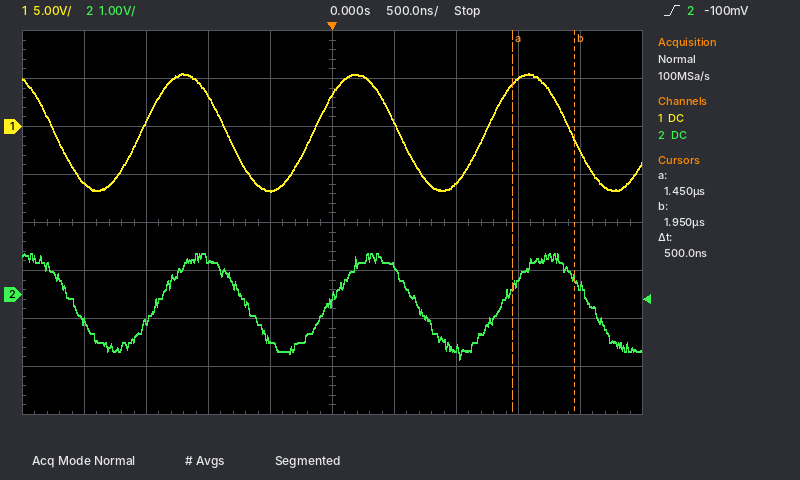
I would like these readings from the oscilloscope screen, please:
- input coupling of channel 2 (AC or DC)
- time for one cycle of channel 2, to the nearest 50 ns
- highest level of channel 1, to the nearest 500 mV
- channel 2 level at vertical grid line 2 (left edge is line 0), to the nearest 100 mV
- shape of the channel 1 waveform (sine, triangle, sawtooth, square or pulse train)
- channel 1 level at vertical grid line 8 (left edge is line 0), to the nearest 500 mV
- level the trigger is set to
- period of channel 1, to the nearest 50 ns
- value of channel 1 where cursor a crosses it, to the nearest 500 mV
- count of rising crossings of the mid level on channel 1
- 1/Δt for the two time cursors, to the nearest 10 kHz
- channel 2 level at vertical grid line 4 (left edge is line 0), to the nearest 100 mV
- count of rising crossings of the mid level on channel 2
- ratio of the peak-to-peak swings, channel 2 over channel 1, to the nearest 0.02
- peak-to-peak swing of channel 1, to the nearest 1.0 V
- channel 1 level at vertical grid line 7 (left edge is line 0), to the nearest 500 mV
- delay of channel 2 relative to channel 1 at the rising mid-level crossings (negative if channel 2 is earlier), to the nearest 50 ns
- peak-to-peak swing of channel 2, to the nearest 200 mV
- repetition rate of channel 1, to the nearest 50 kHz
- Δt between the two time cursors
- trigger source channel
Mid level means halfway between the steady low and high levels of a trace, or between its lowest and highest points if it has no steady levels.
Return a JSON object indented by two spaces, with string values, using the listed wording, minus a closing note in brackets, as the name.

{
  "input coupling of channel 2": "DC",
  "time for one cycle of channel 2, to the nearest 50 ns": "1.40 µs",
  "highest level of channel 1, to the nearest 500 mV": "5.5 V",
  "channel 2 level at vertical grid line 2 (left edge is line 0), to the nearest 100 mV": "-500 mV",
  "shape of the channel 1 waveform": "sine",
  "channel 1 level at vertical grid line 8 (left edge is line 0), to the nearest 500 mV": "5.0 V",
  "level the trigger is set to": "-100 mV",
  "period of channel 1, to the nearest 50 ns": "1.40 µs",
  "value of channel 1 where cursor a crosses it, to the nearest 500 mV": "4.5 V",
  "count of rising crossings of the mid level on channel 1": "3",
  "1/Δt for the two time cursors, to the nearest 10 kHz": "2.00 MHz",
  "channel 2 level at vertical grid line 4 (left edge is line 0), to the nearest 100 mV": "-900 mV",
  "count of rising crossings of the mid level on channel 2": "3",
  "ratio of the peak-to-peak swings, channel 2 over channel 1, to the nearest 0.02": "0.18",
  "peak-to-peak swing of channel 1, to the nearest 1.0 V": "12.0 V",
  "channel 1 level at vertical grid line 7 (left edge is line 0), to the nearest 500 mV": "-6.0 V",
  "delay of channel 2 relative to channel 1 at the rising mid-level crossings (negative if channel 2 is earlier), to the nearest 50 ns": "+100 ns",
  "peak-to-peak swing of channel 2, to the nearest 200 mV": "2.2 V",
  "repetition rate of channel 1, to the nearest 50 kHz": "700 kHz",
  "Δt between the two time cursors": "500 ns",
  "trigger source channel": "channel 2"
}
